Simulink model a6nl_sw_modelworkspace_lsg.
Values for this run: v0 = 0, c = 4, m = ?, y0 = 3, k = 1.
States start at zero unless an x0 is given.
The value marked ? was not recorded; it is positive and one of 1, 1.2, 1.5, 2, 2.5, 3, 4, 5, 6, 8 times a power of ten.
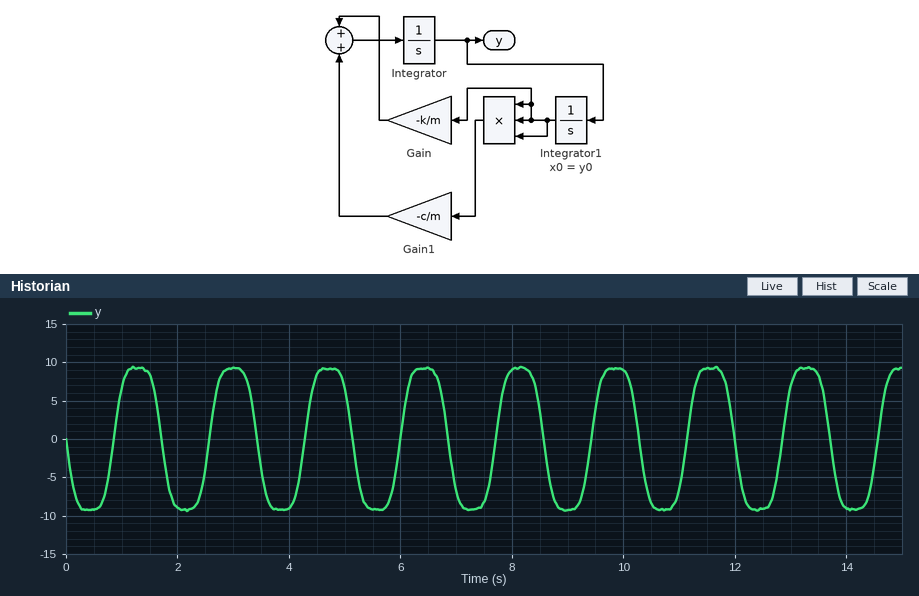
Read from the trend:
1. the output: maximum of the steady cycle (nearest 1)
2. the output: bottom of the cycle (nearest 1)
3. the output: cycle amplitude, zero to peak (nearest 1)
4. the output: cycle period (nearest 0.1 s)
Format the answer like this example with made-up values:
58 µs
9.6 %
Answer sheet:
9
-9
9
1.7 s
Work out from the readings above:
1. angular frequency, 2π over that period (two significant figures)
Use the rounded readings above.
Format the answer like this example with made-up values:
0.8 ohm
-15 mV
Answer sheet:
3.7 rad/s
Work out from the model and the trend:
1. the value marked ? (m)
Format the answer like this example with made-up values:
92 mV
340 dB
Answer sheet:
2
